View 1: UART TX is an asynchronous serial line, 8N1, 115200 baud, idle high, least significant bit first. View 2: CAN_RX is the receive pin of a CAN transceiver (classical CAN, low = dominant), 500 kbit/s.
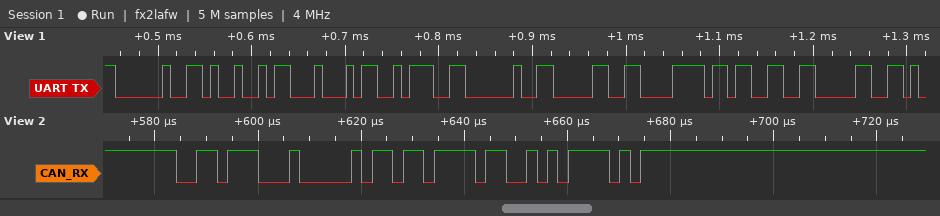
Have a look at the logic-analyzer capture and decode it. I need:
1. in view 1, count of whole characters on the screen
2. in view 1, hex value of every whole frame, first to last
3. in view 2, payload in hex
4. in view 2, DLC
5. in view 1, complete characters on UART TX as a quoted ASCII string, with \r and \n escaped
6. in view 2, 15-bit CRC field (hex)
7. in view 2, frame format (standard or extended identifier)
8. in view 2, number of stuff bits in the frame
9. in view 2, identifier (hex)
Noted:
9
20 49 44 3A 20 30 78 33 30
B7
1
" ID: 0x30"
0x595E
standard
1
0x371
